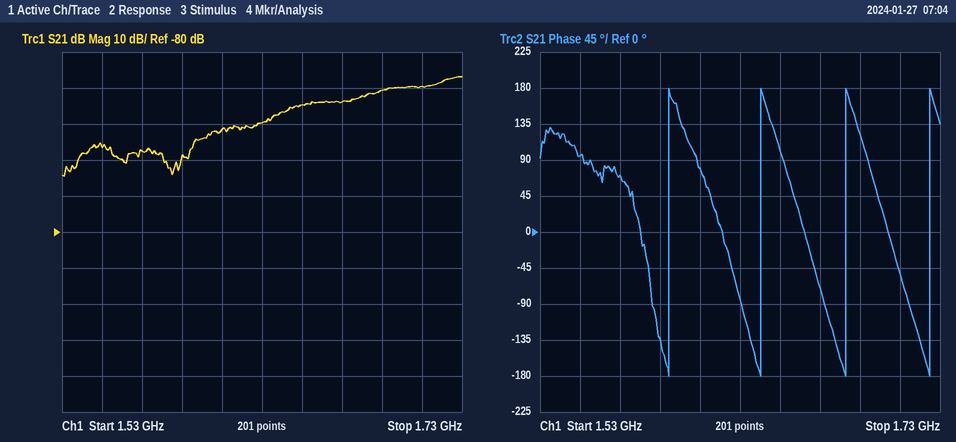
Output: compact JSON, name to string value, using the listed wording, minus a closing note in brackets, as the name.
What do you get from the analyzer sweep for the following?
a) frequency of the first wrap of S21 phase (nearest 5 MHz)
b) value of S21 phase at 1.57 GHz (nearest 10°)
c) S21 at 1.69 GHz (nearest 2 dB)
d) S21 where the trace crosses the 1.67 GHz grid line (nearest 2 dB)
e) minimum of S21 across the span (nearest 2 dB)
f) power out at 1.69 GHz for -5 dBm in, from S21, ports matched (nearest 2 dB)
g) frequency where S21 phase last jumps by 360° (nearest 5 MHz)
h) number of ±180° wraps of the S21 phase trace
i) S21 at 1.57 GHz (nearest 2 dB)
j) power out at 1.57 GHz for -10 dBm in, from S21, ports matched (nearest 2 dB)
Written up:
{"frequency of the first wrap of S21 phase": "1.595 GHz", "value of S21 phase at 1.57 GHz": "70°", "S21 at 1.69 GHz": "-40 dB", "S21 where the trace crosses the 1.67 GHz grid line": "-44 dB", "minimum of S21 across the span": "-64 dB", "power out at 1.69 GHz for -5 dBm in, from S21, ports matched": "-46 dBm", "frequency where S21 phase last jumps by 360°": "1.725 GHz", "number of ±180° wraps of the S21 phase trace": "4", "S21 at 1.57 GHz": "-58 dB", "power out at 1.57 GHz for -10 dBm in, from S21, ports matched": "-68 dBm"}
